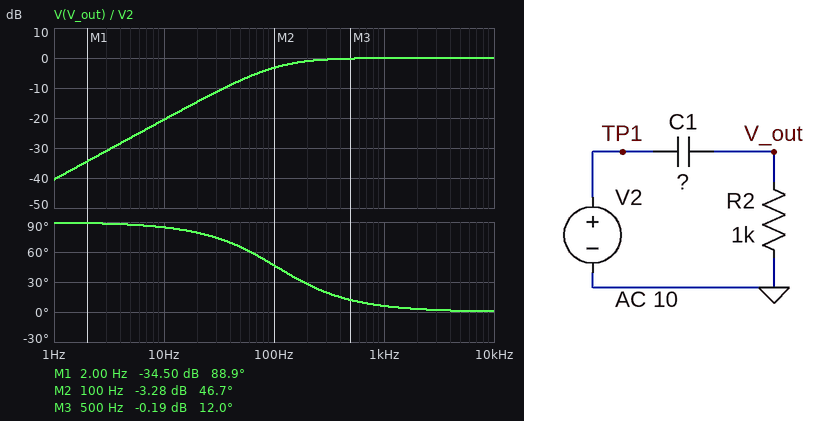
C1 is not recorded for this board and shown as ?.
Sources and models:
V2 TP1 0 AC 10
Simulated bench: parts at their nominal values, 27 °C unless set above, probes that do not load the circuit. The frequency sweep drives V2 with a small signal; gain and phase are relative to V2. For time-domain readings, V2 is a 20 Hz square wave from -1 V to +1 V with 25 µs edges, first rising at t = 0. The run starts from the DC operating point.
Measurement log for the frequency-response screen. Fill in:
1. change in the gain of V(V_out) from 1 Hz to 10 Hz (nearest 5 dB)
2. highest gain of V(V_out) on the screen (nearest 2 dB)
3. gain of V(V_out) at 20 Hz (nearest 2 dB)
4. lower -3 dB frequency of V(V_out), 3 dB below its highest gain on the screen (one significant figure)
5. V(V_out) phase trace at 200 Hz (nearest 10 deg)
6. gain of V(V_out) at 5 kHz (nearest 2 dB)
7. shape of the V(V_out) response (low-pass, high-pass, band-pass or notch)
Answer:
20 dB
0 dB
-14 dB
100 Hz
30 deg
0 dB
high-pass
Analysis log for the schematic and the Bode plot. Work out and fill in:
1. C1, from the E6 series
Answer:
1.5 µF
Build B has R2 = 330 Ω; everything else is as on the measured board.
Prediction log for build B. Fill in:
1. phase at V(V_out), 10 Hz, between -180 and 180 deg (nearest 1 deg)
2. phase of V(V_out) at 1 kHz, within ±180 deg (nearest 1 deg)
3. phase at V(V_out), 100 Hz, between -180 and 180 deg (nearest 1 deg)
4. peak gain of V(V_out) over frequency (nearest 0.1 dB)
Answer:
88 deg
18 deg
73 deg
0 dB
